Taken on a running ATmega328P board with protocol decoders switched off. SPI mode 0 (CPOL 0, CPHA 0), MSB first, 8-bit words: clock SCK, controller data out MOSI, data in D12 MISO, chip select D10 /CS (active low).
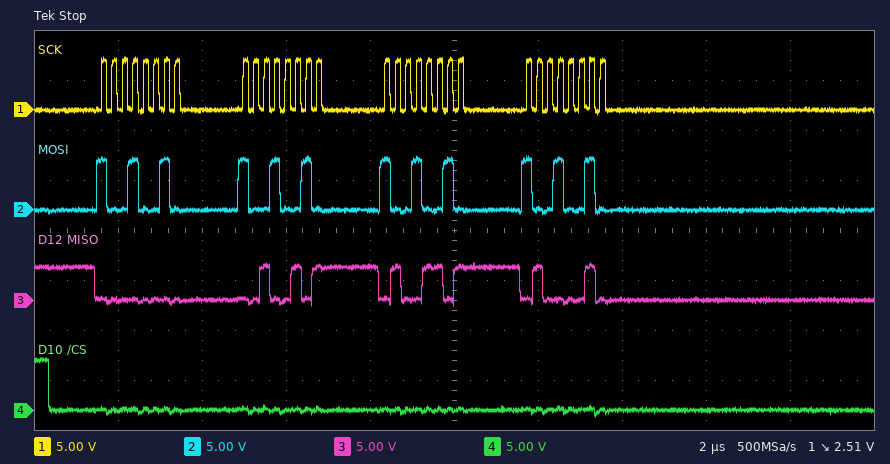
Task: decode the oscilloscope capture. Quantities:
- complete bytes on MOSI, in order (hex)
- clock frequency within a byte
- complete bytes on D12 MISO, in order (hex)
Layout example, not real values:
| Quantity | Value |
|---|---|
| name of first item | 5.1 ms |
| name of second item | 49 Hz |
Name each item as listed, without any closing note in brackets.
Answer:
| Quantity | Value |
|---|---|
| complete bytes on MOSI, in order | 0x92 0x92 0x92 0x92 |
| clock frequency within a byte | 4 MHz |
| complete bytes on D12 MISO, in order | 0x00 0x25 0x4D 0x42 |
